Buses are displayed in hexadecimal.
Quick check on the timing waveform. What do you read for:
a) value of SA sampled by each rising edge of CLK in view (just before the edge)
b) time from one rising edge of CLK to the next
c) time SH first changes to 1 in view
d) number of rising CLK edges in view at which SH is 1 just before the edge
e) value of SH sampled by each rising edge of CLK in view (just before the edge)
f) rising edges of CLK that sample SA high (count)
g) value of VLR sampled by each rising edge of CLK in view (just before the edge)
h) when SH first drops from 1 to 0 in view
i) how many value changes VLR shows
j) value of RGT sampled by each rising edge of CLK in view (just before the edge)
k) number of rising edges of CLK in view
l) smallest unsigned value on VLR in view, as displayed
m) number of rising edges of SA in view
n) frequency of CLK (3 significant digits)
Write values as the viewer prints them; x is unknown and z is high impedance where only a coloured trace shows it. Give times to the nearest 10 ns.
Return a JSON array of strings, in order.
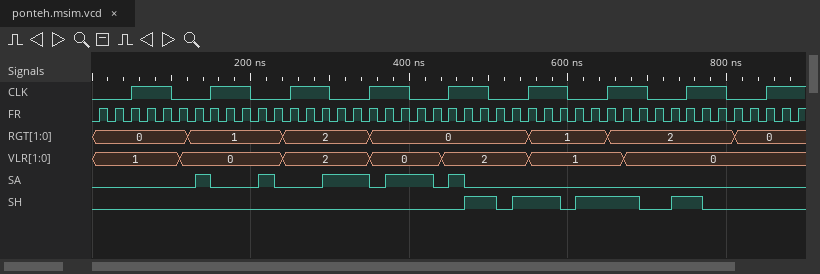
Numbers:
["0 1 0 1 0 0 0 0 0", "100 ns", "470 ns", "3", "0 0 0 0 0 1 1 1 0", "2", "1, 0, 2, 2, 2, 2, 1, 0, 0", "510 ns", "6", "0, 1, 2, 2, 0, 0, 1, 2, 0", "9", "0", "5", "10.0 MHz"]
